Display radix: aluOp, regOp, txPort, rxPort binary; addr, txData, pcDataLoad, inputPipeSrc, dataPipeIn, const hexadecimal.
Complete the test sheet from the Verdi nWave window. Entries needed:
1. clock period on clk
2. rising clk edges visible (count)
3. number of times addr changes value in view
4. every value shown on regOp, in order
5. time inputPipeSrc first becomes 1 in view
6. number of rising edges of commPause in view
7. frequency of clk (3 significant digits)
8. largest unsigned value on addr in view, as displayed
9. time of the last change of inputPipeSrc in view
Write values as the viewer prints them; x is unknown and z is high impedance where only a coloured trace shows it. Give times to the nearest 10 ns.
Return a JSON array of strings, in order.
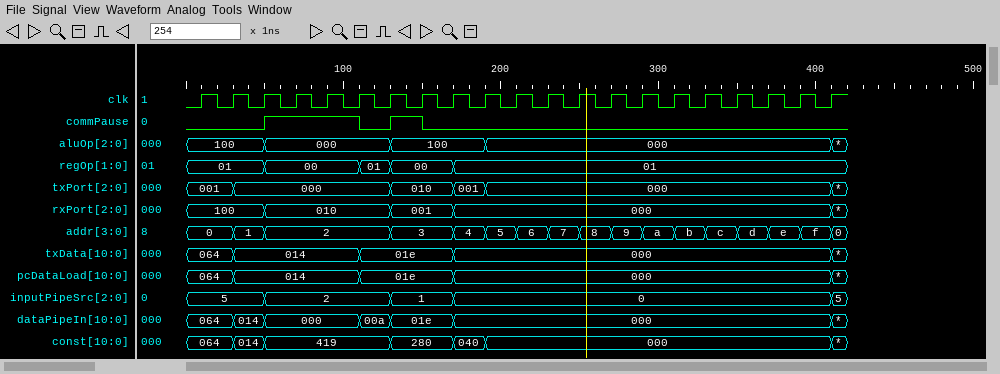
["20 ns", "21", "16", "01, 00, 01, 00, 01", "130 ns", "2", "50.0 MHz", "f", "410 ns"]
